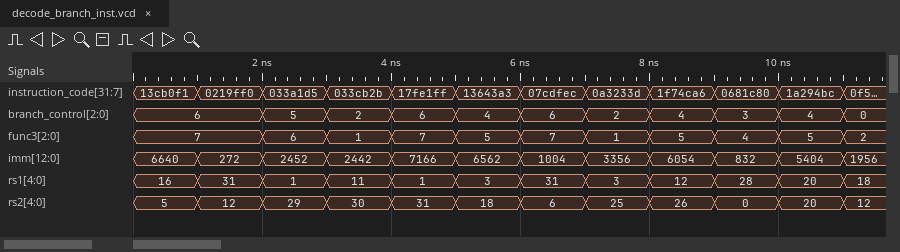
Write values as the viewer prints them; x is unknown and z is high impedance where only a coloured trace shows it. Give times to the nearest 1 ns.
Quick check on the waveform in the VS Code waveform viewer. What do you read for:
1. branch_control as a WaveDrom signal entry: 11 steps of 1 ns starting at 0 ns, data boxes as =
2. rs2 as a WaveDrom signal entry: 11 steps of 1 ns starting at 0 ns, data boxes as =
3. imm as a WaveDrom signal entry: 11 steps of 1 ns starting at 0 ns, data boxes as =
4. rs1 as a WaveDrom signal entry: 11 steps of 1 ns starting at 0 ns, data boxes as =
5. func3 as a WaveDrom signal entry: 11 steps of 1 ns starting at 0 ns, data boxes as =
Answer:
{name: 'branch_control', wave: '=.=========', data: '6 5 2 6 4 6 2 4 3 4'}
{name: 'rs2', wave: '===========', data: '5 12 29 30 31 18 6 25 26 0 20'}
{name: 'imm', wave: '===========', data: '6640 272 2452 2442 7166 6562 1004 3356 6054 832 5404'}
{name: 'rs1', wave: '===========', data: '16 31 1 11 1 3 31 3 12 28 20'}
{name: 'func3', wave: '=.=========', data: '7 6 1 7 5 7 1 5 4 5'}
